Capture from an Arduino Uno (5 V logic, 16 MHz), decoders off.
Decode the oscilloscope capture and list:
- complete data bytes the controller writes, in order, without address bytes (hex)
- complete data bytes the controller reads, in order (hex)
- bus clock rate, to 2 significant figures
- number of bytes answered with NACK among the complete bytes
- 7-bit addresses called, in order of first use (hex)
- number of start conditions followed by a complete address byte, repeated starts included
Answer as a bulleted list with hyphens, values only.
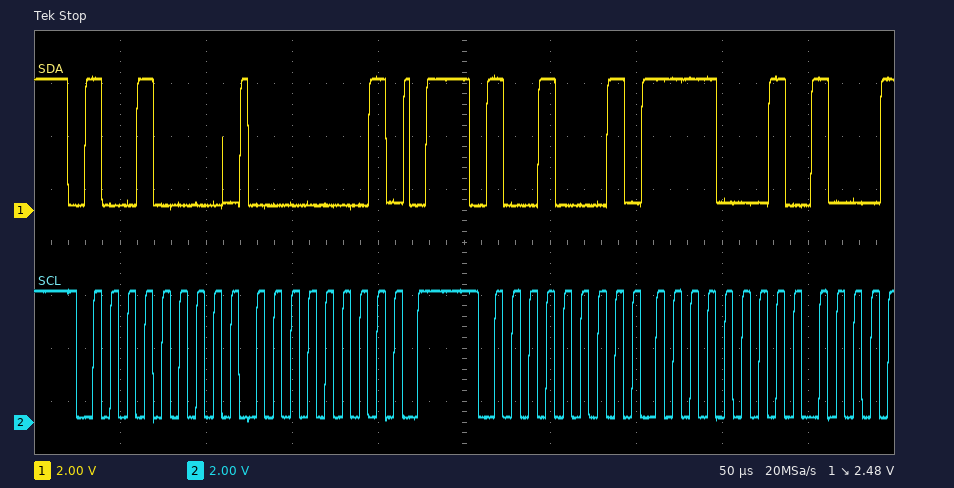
- 01
- F1
- 100 kHz
- 0
- 0x48
- 2
